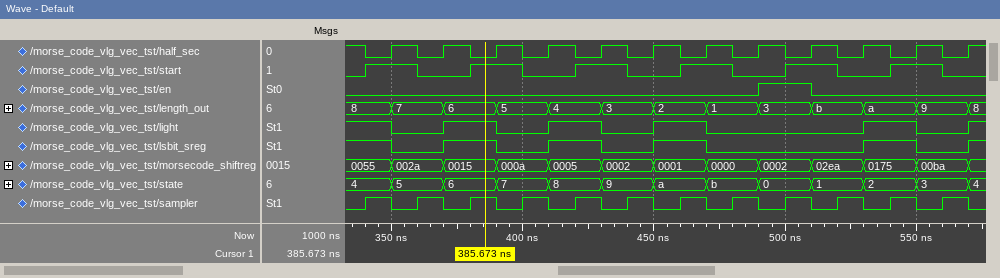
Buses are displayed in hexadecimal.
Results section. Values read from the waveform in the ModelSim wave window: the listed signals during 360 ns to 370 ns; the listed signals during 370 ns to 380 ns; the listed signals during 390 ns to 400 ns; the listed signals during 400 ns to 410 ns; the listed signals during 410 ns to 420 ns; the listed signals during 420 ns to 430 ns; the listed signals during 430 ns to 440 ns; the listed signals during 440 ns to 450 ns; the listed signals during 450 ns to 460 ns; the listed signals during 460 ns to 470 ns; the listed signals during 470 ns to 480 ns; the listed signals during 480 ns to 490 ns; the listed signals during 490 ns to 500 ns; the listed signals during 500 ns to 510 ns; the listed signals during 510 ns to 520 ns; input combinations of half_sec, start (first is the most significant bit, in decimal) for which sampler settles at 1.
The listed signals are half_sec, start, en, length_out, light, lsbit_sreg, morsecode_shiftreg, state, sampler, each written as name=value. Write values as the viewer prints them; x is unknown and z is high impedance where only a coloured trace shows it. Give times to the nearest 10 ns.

half_sec=0, start=0, en=0, length_out=7, light=0, lsbit_sreg=0, morsecode_shiftreg=002a, state=5, sampler=1
half_sec=1, start=0, en=0, length_out=6, light=1, lsbit_sreg=1, morsecode_shiftreg=0015, state=6, sampler=0
half_sec=1, start=1, en=0, length_out=5, light=0, lsbit_sreg=0, morsecode_shiftreg=000a, state=7, sampler=0
half_sec=0, start=0, en=0, length_out=5, light=0, lsbit_sreg=0, morsecode_shiftreg=000a, state=7, sampler=1
half_sec=1, start=0, en=0, length_out=4, light=1, lsbit_sreg=1, morsecode_shiftreg=0005, state=8, sampler=0
half_sec=0, start=1, en=0, length_out=4, light=1, lsbit_sreg=1, morsecode_shiftreg=0005, state=8, sampler=1
half_sec=1, start=1, en=0, length_out=3, light=0, lsbit_sreg=0, morsecode_shiftreg=0002, state=9, sampler=0
half_sec=0, start=0, en=0, length_out=3, light=0, lsbit_sreg=0, morsecode_shiftreg=0002, state=9, sampler=1
half_sec=1, start=0, en=0, length_out=2, light=1, lsbit_sreg=1, morsecode_shiftreg=0001, state=a, sampler=0
half_sec=0, start=1, en=0, length_out=2, light=1, lsbit_sreg=1, morsecode_shiftreg=0001, state=a, sampler=1
half_sec=1, start=1, en=0, length_out=1, light=0, lsbit_sreg=0, morsecode_shiftreg=0000, state=b, sampler=0
half_sec=0, start=0, en=0, length_out=1, light=0, lsbit_sreg=0, morsecode_shiftreg=0000, state=b, sampler=1
half_sec=1, start=0, en=1, length_out=3, light=0, lsbit_sreg=0, morsecode_shiftreg=0002, state=0, sampler=0
half_sec=0, start=1, en=1, length_out=3, light=0, lsbit_sreg=0, morsecode_shiftreg=0002, state=0, sampler=1
half_sec=1, start=1, en=0, length_out=b, light=0, lsbit_sreg=0, morsecode_shiftreg=02ea, state=1, sampler=0
0, 1
